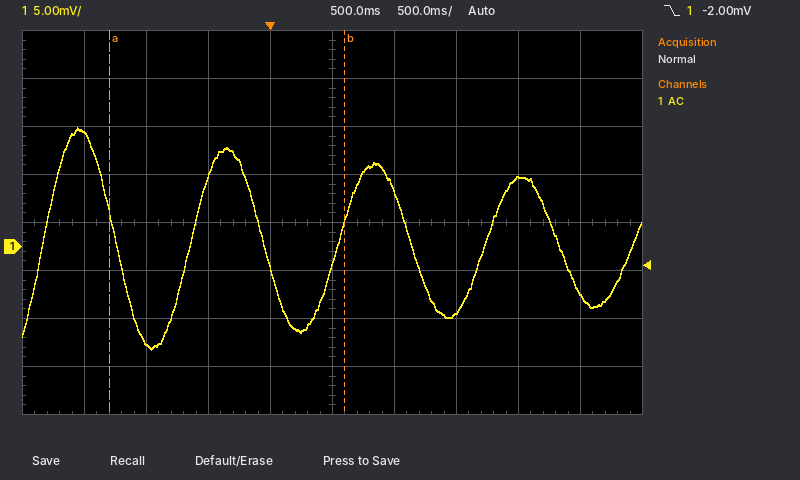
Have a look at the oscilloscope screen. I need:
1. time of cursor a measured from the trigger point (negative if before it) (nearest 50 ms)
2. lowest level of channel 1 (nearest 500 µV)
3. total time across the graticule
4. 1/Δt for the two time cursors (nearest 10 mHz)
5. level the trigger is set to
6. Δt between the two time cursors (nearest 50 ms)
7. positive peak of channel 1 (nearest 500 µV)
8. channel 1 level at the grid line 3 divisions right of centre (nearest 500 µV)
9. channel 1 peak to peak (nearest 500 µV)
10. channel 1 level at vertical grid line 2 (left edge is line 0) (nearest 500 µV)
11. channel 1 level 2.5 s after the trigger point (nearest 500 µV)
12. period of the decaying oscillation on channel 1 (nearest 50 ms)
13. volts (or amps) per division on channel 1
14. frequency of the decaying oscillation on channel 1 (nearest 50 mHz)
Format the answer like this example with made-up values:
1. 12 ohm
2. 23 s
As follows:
1. -1.30 s
2. -10.5 mV
3. 5 s
4. 530 mHz
5. -2.00 mV
6. 1.90 s
7. 12.5 mV
8. 7.0 mV
9. 23.0 mV
10. -10.0 mV
11. -5.0 mV
12. 1.20 s
13. 5 mV
14. 850 mHz
